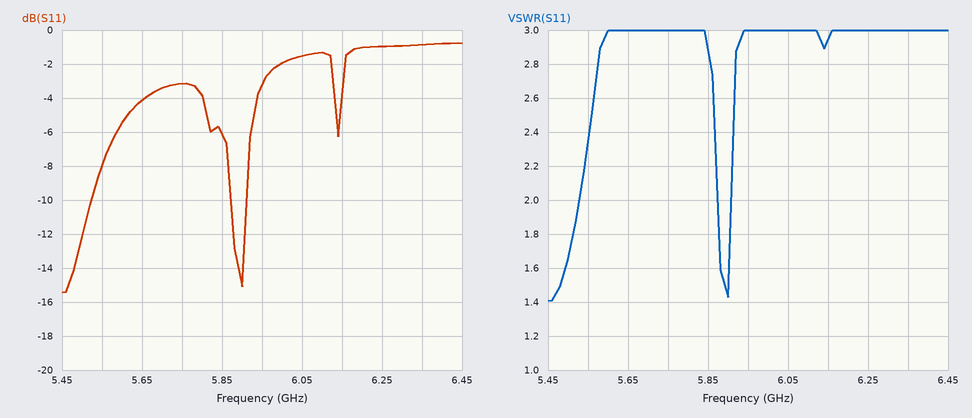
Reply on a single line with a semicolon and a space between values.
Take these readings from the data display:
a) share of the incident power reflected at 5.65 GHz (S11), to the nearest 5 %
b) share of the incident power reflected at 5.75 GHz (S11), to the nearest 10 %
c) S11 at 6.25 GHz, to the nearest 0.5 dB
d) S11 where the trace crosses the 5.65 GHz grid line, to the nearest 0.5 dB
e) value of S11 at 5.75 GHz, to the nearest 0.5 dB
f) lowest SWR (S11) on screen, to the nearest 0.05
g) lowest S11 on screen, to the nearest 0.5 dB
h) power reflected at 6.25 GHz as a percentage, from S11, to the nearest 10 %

40 %; 50 %; -1.0 dB; -4.0 dB; -3.0 dB; 1.40; -15.5 dB; 80 %
